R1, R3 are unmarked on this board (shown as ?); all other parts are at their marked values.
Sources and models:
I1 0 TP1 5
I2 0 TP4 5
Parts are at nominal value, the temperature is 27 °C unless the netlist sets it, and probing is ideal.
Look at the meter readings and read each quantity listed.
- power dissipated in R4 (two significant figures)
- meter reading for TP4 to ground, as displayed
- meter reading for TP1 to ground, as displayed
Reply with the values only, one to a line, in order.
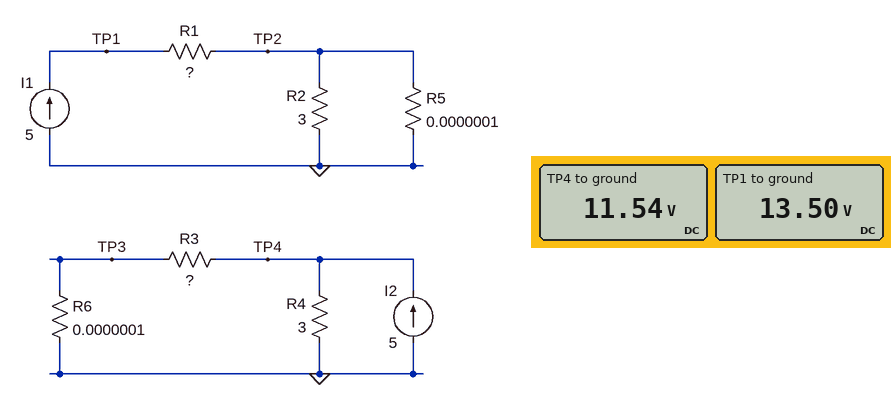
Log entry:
44 W
11.54 V
13.50 V
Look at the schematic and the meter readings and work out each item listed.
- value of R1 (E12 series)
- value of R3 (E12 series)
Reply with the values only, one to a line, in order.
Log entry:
2.7 Ω
10 Ω
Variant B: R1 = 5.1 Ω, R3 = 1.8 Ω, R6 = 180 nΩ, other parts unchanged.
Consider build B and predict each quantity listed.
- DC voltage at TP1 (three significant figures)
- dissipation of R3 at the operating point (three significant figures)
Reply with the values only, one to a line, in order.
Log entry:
25.5 V
17.6 W
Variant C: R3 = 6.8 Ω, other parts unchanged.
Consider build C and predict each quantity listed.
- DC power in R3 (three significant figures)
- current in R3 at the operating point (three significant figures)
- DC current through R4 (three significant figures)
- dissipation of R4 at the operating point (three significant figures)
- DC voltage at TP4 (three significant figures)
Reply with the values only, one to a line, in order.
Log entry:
15.9 W
1.53 A
3.47 A
36.1 W
10.4 V
